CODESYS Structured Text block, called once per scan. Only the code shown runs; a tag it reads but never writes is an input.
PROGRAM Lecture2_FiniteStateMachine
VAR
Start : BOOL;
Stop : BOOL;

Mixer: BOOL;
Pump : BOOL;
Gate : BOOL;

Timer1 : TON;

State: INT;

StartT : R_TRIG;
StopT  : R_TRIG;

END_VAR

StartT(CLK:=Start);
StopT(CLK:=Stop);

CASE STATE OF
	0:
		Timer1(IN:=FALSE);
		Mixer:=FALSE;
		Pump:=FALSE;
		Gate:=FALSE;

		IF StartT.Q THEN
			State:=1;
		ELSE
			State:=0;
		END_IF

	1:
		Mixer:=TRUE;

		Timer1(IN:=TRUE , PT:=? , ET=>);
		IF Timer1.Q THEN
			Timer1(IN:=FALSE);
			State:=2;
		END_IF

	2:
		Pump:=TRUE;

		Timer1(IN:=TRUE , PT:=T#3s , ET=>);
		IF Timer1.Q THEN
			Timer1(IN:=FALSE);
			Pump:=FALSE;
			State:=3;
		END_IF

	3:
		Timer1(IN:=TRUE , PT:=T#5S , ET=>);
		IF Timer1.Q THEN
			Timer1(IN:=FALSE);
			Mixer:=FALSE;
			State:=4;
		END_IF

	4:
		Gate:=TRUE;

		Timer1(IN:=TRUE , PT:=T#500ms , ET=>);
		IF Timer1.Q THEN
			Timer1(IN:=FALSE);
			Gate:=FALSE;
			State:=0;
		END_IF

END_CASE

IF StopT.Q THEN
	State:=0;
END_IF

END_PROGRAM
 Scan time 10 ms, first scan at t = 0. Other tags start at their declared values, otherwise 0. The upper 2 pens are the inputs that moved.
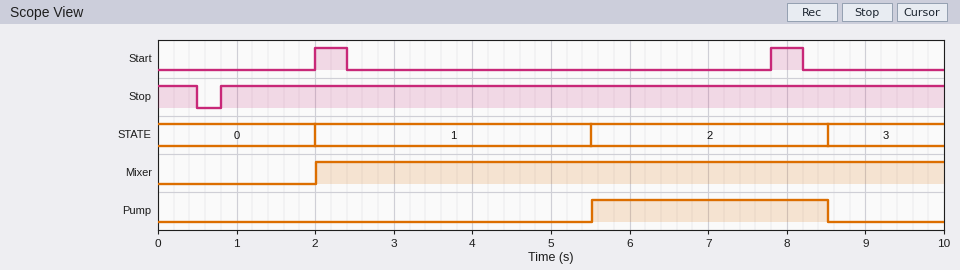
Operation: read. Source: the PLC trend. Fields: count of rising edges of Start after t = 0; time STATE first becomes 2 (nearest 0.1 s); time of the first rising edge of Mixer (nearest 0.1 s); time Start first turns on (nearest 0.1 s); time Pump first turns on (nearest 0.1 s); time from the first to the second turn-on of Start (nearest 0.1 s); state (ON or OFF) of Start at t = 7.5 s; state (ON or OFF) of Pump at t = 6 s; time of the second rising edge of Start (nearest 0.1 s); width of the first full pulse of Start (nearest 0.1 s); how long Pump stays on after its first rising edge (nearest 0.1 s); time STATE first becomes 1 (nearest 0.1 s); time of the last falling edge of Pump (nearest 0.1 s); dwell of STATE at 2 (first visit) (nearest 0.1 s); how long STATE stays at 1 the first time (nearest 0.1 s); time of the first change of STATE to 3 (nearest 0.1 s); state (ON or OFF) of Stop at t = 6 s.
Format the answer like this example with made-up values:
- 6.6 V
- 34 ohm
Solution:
- 2
- 5.5 s
- 2.0 s
- 2.0 s
- 5.5 s
- 5.8 s
- OFF
- ON
- 7.8 s
- 0.4 s
- 3.0 s
- 2.0 s
- 8.5 s
- 3.0 s
- 3.5 s
- 8.5 s
- ON
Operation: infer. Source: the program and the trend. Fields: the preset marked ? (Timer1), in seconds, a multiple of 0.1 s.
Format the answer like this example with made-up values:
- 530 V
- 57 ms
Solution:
- 3.5 s
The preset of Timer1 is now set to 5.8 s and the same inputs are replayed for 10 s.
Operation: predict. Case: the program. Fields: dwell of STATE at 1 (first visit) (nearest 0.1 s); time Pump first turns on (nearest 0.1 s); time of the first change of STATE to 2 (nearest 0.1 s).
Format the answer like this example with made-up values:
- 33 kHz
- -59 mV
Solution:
- 5.8 s
- 7.8 s
- 7.8 s
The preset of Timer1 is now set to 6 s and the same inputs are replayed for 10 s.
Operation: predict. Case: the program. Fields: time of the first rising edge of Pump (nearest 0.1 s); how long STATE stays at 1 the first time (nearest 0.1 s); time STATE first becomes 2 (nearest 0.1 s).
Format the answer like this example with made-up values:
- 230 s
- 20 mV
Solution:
- 8.0 s
- 6.0 s
- 8.0 s
